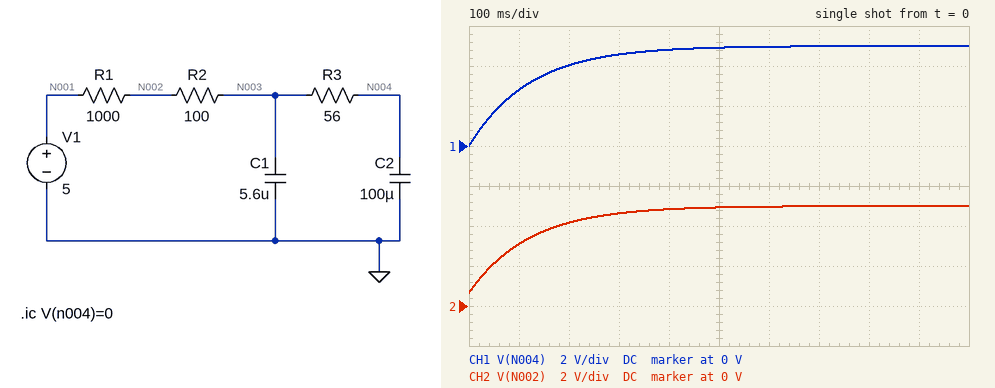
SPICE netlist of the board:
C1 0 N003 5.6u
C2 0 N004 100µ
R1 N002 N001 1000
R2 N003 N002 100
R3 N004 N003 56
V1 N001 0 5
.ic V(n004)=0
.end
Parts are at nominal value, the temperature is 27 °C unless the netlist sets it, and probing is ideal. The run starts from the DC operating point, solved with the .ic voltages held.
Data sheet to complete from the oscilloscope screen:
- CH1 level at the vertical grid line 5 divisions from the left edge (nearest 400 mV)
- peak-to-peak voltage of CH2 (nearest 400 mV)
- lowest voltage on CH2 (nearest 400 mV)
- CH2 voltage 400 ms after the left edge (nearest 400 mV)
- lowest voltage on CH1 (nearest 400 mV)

4.8 V
4.4 V
800 mV
4.8 V
0 V
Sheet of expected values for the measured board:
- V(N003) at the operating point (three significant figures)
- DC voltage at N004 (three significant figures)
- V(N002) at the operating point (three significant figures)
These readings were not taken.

5.00 V
5.00 V
5.00 V
